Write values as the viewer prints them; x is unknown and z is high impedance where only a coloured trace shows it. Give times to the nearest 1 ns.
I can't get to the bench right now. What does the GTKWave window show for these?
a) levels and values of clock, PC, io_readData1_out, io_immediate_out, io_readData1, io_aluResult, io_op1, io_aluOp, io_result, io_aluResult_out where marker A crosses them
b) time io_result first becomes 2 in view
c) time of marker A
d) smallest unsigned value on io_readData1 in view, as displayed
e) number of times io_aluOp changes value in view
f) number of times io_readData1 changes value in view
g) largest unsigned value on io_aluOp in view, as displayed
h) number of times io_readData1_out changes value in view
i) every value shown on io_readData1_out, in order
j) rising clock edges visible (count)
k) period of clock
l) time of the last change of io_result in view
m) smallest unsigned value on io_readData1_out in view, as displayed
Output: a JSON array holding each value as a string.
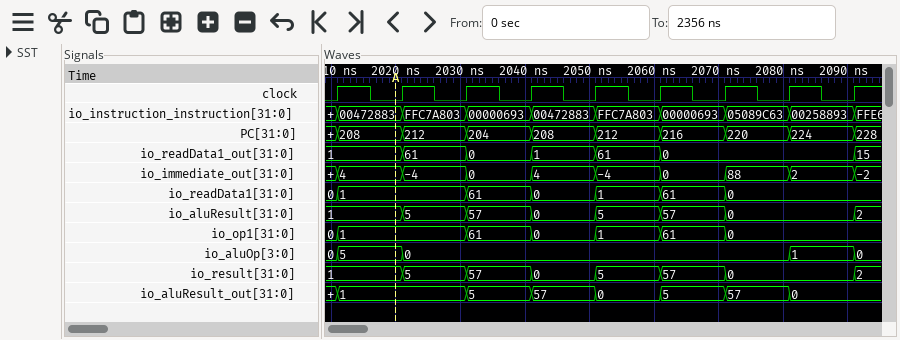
["clock=0, PC=208, io_readData1_out=1, io_immediate_out=4, io_readData1=1, io_aluResult=1, io_op1=1, io_aluOp=5, io_result=1, io_aluResult_out=1", "2091 ns", "2020 ns", "0", "4", "6", "5", "6", "1, 61, 0, 1, 61, 0, 15", "9", "10 ns", "2091 ns", "0"]
